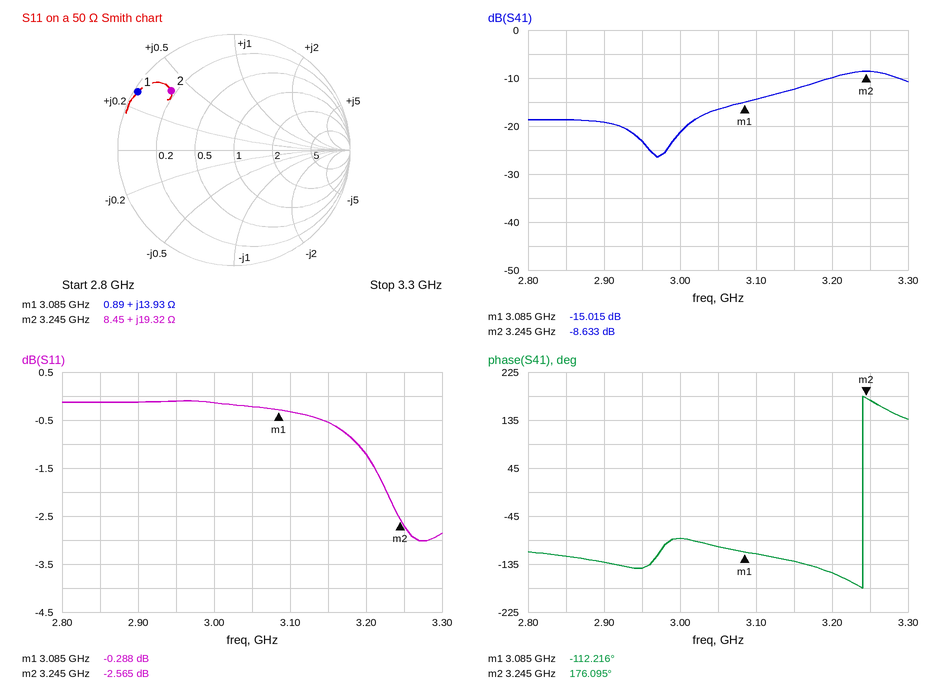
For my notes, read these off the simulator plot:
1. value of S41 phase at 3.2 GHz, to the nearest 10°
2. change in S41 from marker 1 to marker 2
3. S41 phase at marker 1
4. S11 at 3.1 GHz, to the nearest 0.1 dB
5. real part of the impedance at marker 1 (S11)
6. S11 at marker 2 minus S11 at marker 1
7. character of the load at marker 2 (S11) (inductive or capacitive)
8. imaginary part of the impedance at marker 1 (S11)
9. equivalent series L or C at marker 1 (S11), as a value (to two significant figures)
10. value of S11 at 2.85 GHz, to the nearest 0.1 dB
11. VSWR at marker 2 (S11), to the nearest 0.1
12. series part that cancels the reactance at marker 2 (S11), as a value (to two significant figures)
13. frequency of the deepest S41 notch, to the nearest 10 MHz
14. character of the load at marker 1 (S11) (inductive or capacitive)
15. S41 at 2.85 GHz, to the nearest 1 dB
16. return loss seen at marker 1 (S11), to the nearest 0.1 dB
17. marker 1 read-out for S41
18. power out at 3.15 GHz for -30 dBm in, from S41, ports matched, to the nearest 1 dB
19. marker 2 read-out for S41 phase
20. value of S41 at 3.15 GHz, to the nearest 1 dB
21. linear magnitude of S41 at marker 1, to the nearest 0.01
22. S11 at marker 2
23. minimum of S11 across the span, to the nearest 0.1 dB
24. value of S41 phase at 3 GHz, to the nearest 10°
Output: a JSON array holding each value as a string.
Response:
["-150°", "6.382 dB", "-112.216°", "-0.3 dB", "0.89 Ω", "-2.277 dB", "inductive", "+13.93 Ω", "720 pH", "-0.1 dB", "6.8", "2.5 pF", "2.97 GHz", "inductive", "-19 dB", "0.3 dB", "-15.015 dB", "-42 dBm", "176.095°", "-12 dB", "0.18", "-2.565 dB", "-3.0 dB", "-90°"]
